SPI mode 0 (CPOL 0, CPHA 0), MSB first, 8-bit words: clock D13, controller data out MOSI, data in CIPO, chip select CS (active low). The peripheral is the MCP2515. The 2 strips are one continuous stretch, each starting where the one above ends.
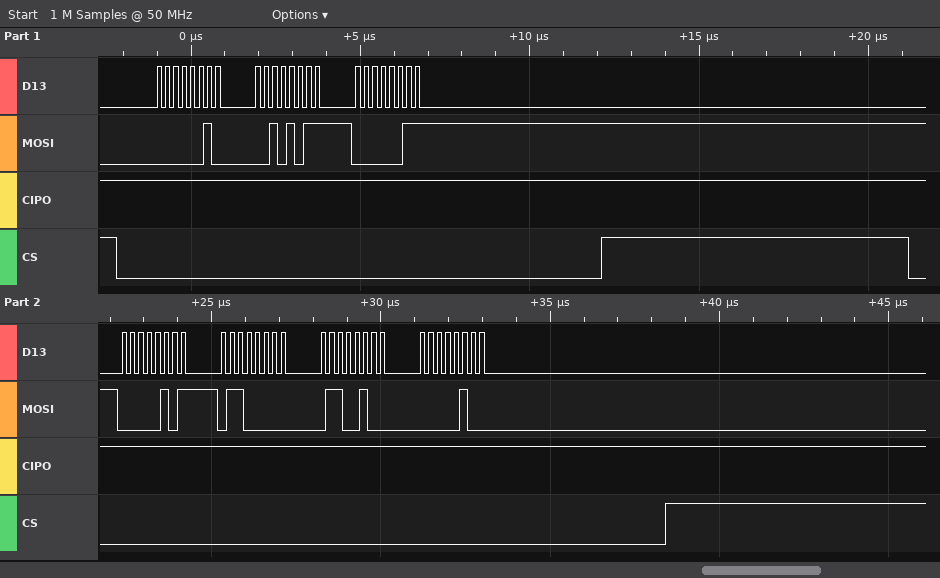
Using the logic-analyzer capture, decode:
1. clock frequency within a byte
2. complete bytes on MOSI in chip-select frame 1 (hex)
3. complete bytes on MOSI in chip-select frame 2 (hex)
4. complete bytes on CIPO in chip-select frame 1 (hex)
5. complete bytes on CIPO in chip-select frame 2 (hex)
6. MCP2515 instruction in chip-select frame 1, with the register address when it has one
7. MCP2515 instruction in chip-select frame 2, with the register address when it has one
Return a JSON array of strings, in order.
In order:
["4 MHz", "02 2B 03", "05 60 64 04", "FF FF FF", "FF FF FF FF", "WRITE 0x2B", "BIT MODIFY 0x60"]
